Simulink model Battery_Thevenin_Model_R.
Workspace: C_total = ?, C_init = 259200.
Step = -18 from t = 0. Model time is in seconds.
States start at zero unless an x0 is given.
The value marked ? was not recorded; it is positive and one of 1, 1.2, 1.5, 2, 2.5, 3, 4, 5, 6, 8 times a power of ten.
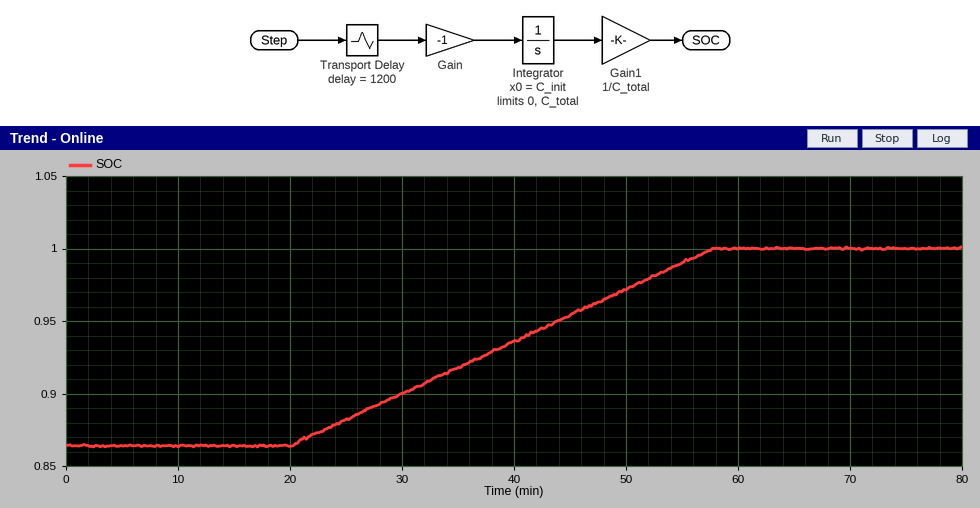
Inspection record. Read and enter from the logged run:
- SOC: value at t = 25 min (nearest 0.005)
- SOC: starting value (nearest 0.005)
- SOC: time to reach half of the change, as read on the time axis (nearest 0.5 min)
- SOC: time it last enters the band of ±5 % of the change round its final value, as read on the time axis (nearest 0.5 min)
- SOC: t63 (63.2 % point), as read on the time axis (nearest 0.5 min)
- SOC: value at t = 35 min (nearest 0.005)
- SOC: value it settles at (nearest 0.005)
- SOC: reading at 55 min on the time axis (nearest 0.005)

0.880
0.865
39.0 min
56.0 min
44.0 min
0.920
1.000
0.990
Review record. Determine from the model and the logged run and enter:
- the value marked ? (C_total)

300000
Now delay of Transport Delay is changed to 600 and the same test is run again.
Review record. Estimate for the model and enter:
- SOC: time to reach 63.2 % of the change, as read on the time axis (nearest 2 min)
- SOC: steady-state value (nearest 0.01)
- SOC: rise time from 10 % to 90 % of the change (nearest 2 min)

34 min
1.00
30 min
